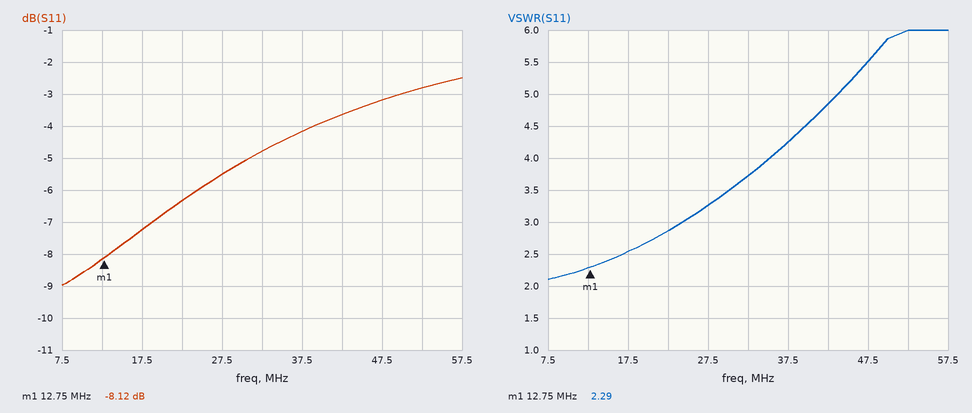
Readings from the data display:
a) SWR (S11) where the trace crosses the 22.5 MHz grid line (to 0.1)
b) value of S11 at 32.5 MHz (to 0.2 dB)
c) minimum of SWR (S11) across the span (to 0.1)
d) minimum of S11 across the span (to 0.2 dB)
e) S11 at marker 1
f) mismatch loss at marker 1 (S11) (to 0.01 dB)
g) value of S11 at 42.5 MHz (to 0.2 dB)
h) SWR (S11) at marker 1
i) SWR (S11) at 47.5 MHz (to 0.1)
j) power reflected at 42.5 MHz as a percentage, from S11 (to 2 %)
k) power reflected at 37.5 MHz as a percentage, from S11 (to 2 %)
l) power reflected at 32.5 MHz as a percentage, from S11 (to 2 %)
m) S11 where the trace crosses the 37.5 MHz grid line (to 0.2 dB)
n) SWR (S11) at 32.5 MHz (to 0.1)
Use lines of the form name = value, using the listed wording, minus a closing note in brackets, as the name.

SWR (S11) where the trace crosses the 22.5 MHz grid line = 2.9
value of S11 at 32.5 MHz = -4.8 dB
minimum of SWR (S11) across the span = 2.1
minimum of S11 across the span = -9.0 dB
S11 at marker 1 = -8.12 dB
mismatch loss at marker 1 (S11) = 0.73 dB
value of S11 at 42.5 MHz = -3.6 dB
SWR (S11) at marker 1 = 2.29
SWR (S11) at 47.5 MHz = 5.5
power reflected at 42.5 MHz as a percentage, from S11 = 44 %
power reflected at 37.5 MHz as a percentage, from S11 = 38 %
power reflected at 32.5 MHz as a percentage, from S11 = 34 %
S11 where the trace crosses the 37.5 MHz grid line = -4.2 dB
SWR (S11) at 32.5 MHz = 3.7
